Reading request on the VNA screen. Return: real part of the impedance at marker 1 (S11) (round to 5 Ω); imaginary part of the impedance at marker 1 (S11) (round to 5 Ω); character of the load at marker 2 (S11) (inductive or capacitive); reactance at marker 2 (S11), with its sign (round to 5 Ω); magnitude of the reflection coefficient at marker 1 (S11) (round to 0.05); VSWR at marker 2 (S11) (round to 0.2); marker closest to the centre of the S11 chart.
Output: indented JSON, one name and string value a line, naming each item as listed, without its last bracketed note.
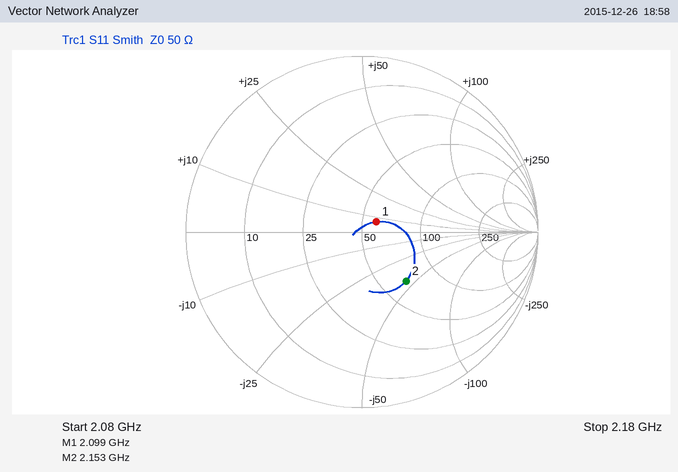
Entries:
{
  "real part of the impedance at marker 1 (S11)": "60 Ω",
  "imaginary part of the impedance at marker 1 (S11)": "+5 Ω",
  "character of the load at marker 2 (S11)": "capacitive",
  "reactance at marker 2 (S11), with its sign": "-45 Ω",
  "magnitude of the reflection coefficient at marker 1 (S11)": "0.10",
  "VSWR at marker 2 (S11)": "2.2",
  "marker closest to the centre of the S11 chart": "marker 1"
}
